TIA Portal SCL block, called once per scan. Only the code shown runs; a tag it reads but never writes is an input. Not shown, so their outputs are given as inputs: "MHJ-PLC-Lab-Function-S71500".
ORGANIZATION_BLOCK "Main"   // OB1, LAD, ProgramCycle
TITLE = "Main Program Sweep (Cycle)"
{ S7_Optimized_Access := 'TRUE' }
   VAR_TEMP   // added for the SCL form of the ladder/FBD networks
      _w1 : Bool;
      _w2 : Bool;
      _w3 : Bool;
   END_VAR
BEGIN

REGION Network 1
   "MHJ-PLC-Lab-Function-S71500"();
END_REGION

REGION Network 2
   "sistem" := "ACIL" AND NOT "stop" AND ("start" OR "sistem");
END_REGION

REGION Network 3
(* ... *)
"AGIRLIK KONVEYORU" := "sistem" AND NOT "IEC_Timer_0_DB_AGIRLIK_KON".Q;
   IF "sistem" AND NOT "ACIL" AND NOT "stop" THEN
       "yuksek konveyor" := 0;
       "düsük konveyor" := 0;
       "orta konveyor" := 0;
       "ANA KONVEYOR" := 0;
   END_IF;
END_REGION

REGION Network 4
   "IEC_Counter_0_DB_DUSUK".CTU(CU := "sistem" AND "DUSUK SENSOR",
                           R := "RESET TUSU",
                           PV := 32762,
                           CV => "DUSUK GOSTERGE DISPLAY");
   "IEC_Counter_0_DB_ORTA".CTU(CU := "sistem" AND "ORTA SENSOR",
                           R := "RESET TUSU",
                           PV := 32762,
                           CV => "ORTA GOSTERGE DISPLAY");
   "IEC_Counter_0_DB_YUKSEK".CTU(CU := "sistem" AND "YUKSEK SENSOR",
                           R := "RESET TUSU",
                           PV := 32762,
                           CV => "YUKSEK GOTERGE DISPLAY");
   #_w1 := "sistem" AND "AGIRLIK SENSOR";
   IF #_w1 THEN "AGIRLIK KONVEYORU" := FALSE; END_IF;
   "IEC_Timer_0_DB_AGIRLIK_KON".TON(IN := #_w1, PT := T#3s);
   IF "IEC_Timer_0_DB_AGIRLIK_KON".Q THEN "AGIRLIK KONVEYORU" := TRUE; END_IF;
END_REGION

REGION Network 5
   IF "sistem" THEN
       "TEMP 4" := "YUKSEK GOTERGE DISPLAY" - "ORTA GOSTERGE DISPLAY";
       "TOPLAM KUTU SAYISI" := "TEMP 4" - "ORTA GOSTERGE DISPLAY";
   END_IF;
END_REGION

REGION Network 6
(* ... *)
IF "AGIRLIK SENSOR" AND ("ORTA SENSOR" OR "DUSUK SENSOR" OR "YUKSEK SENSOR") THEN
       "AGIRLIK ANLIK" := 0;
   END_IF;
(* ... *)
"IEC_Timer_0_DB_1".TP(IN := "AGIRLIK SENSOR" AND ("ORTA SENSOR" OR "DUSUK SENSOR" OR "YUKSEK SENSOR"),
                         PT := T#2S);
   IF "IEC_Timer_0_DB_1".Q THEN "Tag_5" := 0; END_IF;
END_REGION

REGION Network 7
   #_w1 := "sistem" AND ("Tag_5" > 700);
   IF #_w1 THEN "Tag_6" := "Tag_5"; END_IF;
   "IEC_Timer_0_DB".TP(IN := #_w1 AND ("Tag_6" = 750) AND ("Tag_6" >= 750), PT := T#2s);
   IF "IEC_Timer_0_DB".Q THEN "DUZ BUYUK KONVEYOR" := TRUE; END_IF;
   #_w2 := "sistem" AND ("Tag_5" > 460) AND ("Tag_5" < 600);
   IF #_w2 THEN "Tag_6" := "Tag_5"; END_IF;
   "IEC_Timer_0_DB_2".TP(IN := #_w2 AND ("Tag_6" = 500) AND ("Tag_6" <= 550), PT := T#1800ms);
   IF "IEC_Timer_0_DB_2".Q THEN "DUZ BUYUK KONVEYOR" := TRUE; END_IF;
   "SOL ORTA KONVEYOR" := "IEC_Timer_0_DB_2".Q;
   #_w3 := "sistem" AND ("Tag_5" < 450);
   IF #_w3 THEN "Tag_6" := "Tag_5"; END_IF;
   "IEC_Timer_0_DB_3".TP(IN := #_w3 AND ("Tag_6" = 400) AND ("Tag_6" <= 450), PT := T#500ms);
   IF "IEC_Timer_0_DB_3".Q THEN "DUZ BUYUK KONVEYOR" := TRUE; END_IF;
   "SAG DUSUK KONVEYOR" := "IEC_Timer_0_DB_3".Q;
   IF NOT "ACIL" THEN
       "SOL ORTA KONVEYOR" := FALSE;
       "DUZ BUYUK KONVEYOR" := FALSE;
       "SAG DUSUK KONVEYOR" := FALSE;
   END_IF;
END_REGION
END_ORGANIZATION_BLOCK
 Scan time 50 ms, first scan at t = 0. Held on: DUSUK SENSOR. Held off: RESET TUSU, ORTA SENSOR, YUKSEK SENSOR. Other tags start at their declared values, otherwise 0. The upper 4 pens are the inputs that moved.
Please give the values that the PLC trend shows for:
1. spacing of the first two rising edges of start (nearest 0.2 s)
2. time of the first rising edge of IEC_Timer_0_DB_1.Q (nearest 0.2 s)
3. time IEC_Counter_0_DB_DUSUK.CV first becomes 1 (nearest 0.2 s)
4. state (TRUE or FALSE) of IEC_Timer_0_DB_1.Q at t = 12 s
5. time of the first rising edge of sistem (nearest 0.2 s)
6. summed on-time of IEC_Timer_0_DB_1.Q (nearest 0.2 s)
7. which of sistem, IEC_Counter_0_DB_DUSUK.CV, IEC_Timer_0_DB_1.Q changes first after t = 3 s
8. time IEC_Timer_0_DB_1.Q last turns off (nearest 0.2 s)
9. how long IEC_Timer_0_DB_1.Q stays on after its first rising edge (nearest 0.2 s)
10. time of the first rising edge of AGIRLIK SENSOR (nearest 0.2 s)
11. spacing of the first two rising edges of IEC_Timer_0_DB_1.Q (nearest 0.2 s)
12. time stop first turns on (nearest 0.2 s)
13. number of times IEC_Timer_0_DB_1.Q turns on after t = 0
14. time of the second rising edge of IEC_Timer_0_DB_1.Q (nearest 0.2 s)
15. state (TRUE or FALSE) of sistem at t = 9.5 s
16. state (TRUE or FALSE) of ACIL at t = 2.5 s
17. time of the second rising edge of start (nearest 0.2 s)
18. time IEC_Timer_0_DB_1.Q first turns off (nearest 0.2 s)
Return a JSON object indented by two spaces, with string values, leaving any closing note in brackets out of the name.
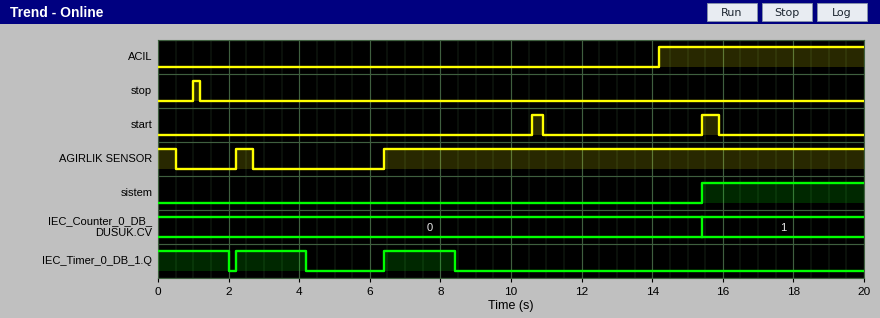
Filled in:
{
  "spacing of the first two rising edges of start": "4.8 s",
  "time of the first rising edge of IEC_Timer_0_DB_1.Q": "2.2 s",
  "time IEC_Counter_0_DB_DUSUK.CV first becomes 1": "15.4 s",
  "state (TRUE or FALSE) of IEC_Timer_0_DB_1.Q at t = 12 s": "FALSE",
  "time of the first rising edge of sistem": "15.4 s",
  "summed on-time of IEC_Timer_0_DB_1.Q": "6.0 s",
  "which of sistem, IEC_Counter_0_DB_DUSUK.CV, IEC_Timer_0_DB_1.Q changes first after t = 3 s": "IEC_Timer_0_DB_1.Q",
  "time IEC_Timer_0_DB_1.Q last turns off": "8.4 s",
  "how long IEC_Timer_0_DB_1.Q stays on after its first rising edge": "2.0 s",
  "time of the first rising edge of AGIRLIK SENSOR": "2.2 s",
  "spacing of the first two rising edges of IEC_Timer_0_DB_1.Q": "4.2 s",
  "time stop first turns on": "1.0 s",
  "number of times IEC_Timer_0_DB_1.Q turns on after t = 0": "2",
  "time of the second rising edge of IEC_Timer_0_DB_1.Q": "6.4 s",
  "state (TRUE or FALSE) of sistem at t = 9.5 s": "FALSE",
  "state (TRUE or FALSE) of ACIL at t = 2.5 s": "FALSE",
  "time of the second rising edge of start": "15.4 s",
  "time IEC_Timer_0_DB_1.Q first turns off": "2.0 s"
}
